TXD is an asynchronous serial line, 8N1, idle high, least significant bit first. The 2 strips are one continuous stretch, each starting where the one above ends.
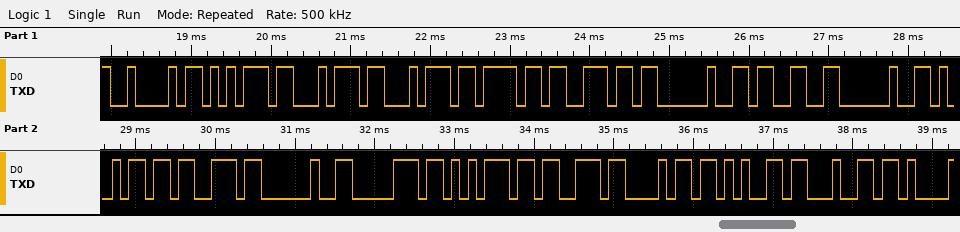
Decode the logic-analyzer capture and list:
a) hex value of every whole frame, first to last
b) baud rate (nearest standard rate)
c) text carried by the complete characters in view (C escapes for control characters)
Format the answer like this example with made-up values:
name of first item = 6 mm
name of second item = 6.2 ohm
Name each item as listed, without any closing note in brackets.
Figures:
hex value of every whole frame, first to last = 0x42 0x75 0x74 0x74 0x6F 0x6E 0x20 0x33 0x20 0x69 0x73 0x20 0x70 0x75 0x73 0x68 0x65 0x64
baud rate = 9600 baud
text carried by the complete characters in view = "Button 3 is pushed"
